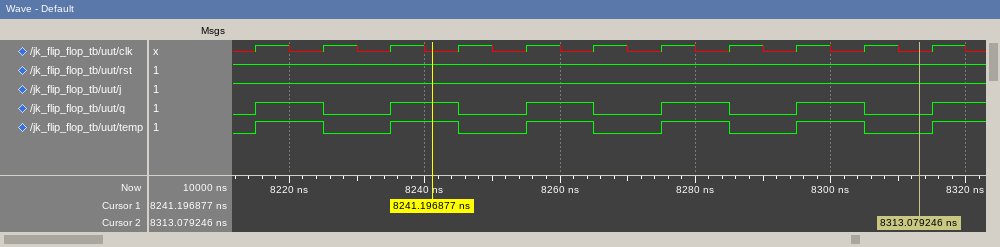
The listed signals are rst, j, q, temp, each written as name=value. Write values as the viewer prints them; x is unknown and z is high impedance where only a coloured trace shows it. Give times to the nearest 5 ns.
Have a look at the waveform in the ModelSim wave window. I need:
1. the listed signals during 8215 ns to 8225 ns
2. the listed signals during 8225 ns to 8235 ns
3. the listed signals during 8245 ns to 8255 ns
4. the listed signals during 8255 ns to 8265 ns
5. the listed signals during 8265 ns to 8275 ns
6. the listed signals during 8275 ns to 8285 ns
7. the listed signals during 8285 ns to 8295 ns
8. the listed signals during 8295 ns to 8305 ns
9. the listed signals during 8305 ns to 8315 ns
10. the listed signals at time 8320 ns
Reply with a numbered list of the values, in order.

1. rst=1, j=1, q=1, temp=1
2. rst=1, j=1, q=0, temp=0
3. rst=1, j=1, q=0, temp=0
4. rst=1, j=1, q=1, temp=1
5. rst=1, j=1, q=0, temp=0
6. rst=1, j=1, q=1, temp=1
7. rst=1, j=1, q=0, temp=0
8. rst=1, j=1, q=1, temp=1
9. rst=1, j=1, q=0, temp=0
10. rst=1, j=1, q=1, temp=1
